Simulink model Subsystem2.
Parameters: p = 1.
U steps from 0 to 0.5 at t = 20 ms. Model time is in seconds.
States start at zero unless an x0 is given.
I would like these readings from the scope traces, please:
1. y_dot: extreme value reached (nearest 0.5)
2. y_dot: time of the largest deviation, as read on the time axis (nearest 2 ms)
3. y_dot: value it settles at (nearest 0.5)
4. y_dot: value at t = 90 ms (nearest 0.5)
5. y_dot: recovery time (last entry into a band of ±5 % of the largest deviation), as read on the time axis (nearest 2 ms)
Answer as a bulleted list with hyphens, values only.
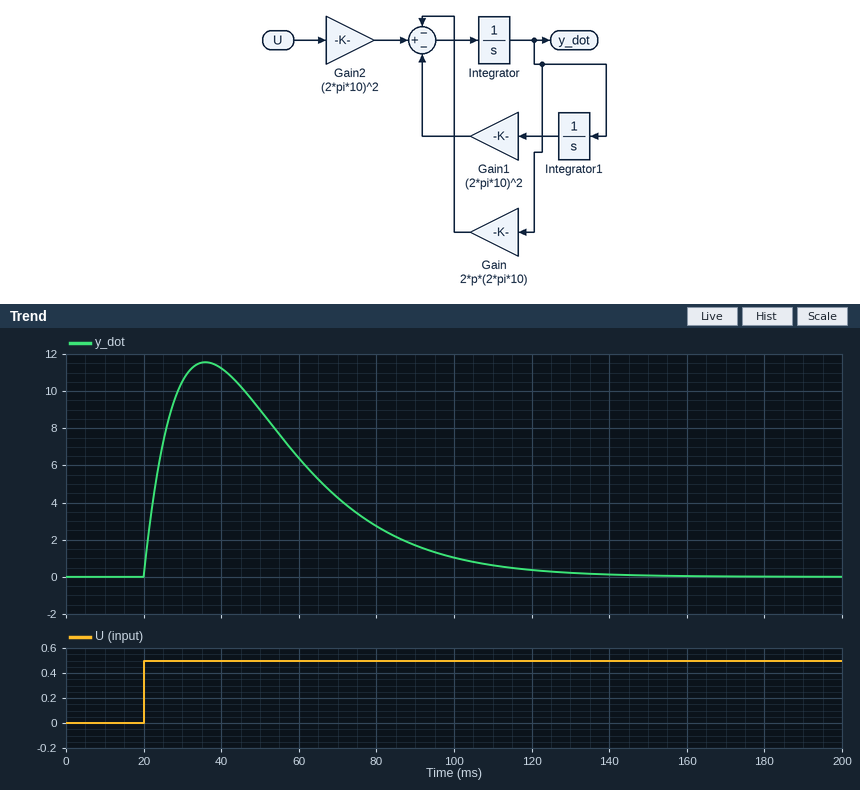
- 11.5
- 36 ms
- 0.0
- 1.5
- 112 ms
